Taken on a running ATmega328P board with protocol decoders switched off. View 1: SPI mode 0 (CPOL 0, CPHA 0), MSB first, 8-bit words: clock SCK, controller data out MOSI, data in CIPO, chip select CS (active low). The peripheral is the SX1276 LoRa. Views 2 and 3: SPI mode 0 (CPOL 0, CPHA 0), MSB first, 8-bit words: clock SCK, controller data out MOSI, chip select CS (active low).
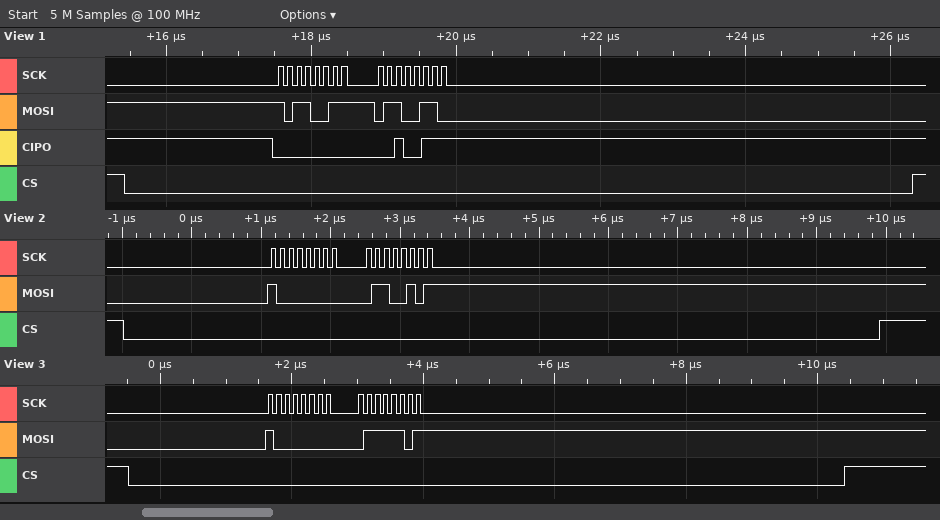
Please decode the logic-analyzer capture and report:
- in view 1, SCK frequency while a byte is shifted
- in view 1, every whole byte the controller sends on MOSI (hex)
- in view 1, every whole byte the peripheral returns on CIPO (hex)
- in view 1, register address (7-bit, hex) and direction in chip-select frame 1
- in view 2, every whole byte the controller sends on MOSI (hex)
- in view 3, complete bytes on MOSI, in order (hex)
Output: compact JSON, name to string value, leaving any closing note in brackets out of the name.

{"in view 1, SCK frequency while a byte is shifted": "8 MHz", "in view 1, every whole byte the controller sends on MOSI": "B3 66", "in view 1, every whole byte the peripheral returns on CIPO": "00 27", "in view 1, register address (7-bit, hex) and direction in chip-select frame 1": "0x33 write", "in view 2, every whole byte the controller sends on MOSI": "0x80 0x65", "in view 3, complete bytes on MOSI, in order": "80 7D"}
